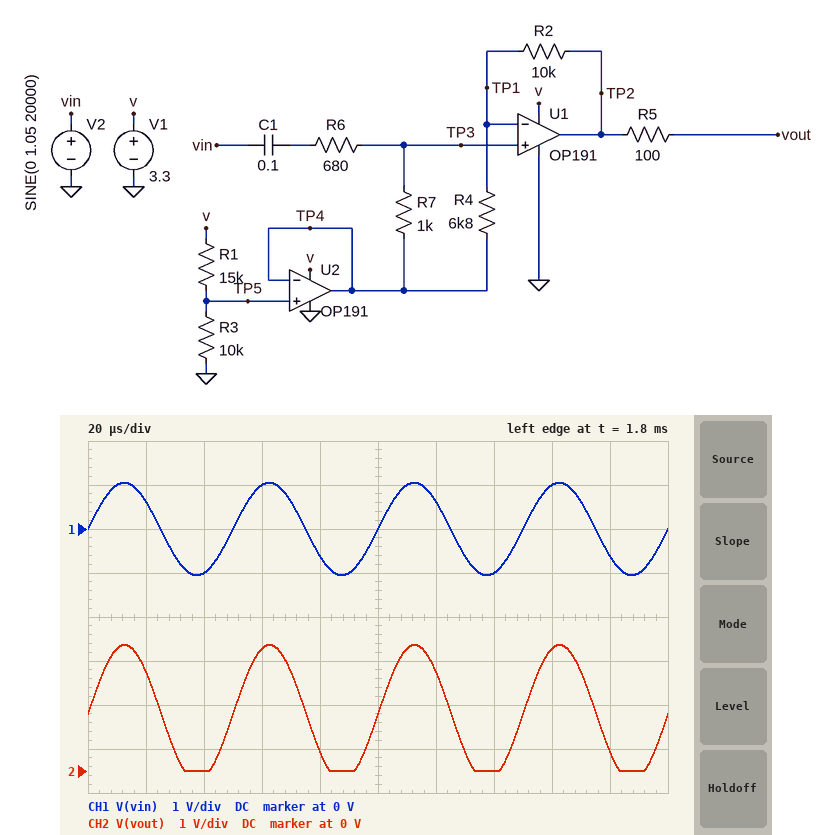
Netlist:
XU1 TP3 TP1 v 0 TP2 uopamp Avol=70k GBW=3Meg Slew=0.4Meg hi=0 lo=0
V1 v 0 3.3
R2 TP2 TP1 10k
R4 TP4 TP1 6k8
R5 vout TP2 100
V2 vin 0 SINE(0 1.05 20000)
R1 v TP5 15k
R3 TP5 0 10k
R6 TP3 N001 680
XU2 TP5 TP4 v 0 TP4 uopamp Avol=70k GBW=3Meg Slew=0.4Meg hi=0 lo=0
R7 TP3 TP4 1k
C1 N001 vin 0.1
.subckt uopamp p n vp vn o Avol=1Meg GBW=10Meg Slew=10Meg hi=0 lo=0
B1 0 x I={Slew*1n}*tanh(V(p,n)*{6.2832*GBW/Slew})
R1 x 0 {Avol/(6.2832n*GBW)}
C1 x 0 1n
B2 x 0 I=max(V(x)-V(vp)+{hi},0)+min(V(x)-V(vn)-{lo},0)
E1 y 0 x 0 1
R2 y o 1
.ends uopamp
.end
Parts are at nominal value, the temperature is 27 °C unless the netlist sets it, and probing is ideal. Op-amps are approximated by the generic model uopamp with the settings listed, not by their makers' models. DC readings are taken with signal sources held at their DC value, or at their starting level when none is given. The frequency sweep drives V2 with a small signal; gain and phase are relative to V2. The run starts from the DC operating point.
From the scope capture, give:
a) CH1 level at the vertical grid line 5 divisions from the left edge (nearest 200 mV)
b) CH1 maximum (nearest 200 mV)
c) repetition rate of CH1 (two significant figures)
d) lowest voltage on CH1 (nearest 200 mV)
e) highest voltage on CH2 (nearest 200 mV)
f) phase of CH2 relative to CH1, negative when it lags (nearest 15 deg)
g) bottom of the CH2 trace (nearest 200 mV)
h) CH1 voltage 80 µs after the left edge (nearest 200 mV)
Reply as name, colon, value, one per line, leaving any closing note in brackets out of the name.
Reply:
CH1 level at the vertical grid line 5 divisions from the left edge: 0 V
CH1 maximum: 1.0 V
repetition rate of CH1: 20 kHz
lowest voltage on CH1: -1.0 V
highest voltage on CH2: 2.8 V
phase of CH2 relative to CH1, negative when it lags: 0 deg
bottom of the CH2 trace: 0 V
CH1 voltage 80 µs after the left edge: -600 mV
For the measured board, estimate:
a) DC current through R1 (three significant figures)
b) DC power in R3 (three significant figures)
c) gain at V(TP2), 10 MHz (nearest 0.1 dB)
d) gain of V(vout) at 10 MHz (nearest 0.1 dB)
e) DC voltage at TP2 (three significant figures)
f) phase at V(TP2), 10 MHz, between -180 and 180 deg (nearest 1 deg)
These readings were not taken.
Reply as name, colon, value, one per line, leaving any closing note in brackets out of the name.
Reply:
DC current through R1: 132 µA
DC power in R3: 174 µW
gain at V(TP2), 10 MHz: -15.0 dB
gain of V(vout) at 10 MHz: -15.0 dB
DC voltage at TP2: 1.32 V
phase at V(TP2), 10 MHz, between -180 and 180 deg: -83 deg
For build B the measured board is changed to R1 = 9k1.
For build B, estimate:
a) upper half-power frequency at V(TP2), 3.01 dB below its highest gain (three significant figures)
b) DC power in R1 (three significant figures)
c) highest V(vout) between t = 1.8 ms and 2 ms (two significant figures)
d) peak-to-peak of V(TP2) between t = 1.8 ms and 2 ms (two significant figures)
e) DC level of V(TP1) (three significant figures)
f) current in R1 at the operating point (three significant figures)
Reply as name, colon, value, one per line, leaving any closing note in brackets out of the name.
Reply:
upper half-power frequency at V(TP2), 3.01 dB below its highest gain: 1.21 MHz
DC power in R1: 272 µW
highest V(vout) between t = 1.8 ms and 2 ms: 3.3 V
peak-to-peak of V(TP2) between t = 1.8 ms and 2 ms: 3.1 V
DC level of V(TP1): 1.73 V
current in R1 at the operating point: 173 µA
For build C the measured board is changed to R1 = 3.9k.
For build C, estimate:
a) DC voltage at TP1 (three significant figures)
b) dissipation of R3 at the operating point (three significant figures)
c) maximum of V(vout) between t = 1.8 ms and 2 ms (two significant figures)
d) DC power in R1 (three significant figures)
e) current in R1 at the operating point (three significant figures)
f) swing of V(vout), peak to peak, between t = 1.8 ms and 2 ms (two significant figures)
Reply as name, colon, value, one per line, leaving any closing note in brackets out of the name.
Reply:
DC voltage at TP1: 2.37 V
dissipation of R3 at the operating point: 564 µW
maximum of V(vout) between t = 1.8 ms and 2 ms: 3.3 V
DC power in R1: 220 µW
current in R1 at the operating point: 237 µA
swing of V(vout), peak to peak, between t = 1.8 ms and 2 ms: 2.5 V
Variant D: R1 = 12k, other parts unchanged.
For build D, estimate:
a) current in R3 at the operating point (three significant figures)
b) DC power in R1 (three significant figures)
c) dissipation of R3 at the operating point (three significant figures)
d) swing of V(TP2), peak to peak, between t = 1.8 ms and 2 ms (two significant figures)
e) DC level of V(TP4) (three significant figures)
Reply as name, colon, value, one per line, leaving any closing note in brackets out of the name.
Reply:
current in R3 at the operating point: 150 µA
DC power in R1: 270 µW
dissipation of R3 at the operating point: 225 µW
swing of V(TP2), peak to peak, between t = 1.8 ms and 2 ms: 3.0 V
DC level of V(TP4): 1.50 V
